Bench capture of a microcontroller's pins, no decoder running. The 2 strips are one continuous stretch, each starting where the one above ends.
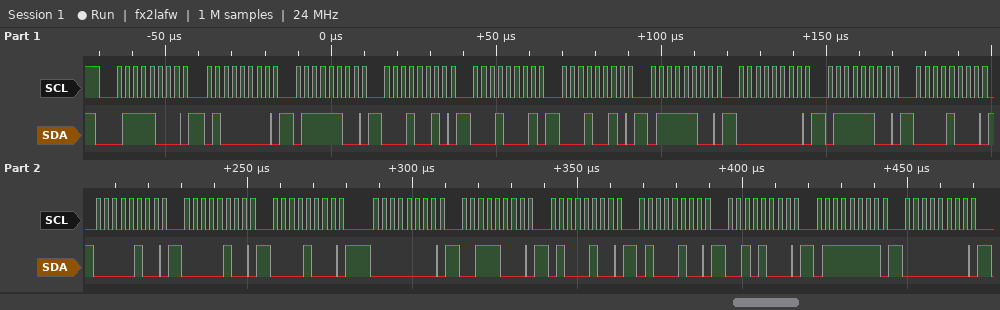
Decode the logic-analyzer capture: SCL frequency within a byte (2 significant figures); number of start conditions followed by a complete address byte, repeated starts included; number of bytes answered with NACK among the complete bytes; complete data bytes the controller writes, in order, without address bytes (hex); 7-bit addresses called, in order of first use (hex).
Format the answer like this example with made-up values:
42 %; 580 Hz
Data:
400 kHz; 1; 0; 40 7C 12 11 12 7C 00 7C 08 04 04 08 00 38 44 44 28 7F 00; 0x3C
